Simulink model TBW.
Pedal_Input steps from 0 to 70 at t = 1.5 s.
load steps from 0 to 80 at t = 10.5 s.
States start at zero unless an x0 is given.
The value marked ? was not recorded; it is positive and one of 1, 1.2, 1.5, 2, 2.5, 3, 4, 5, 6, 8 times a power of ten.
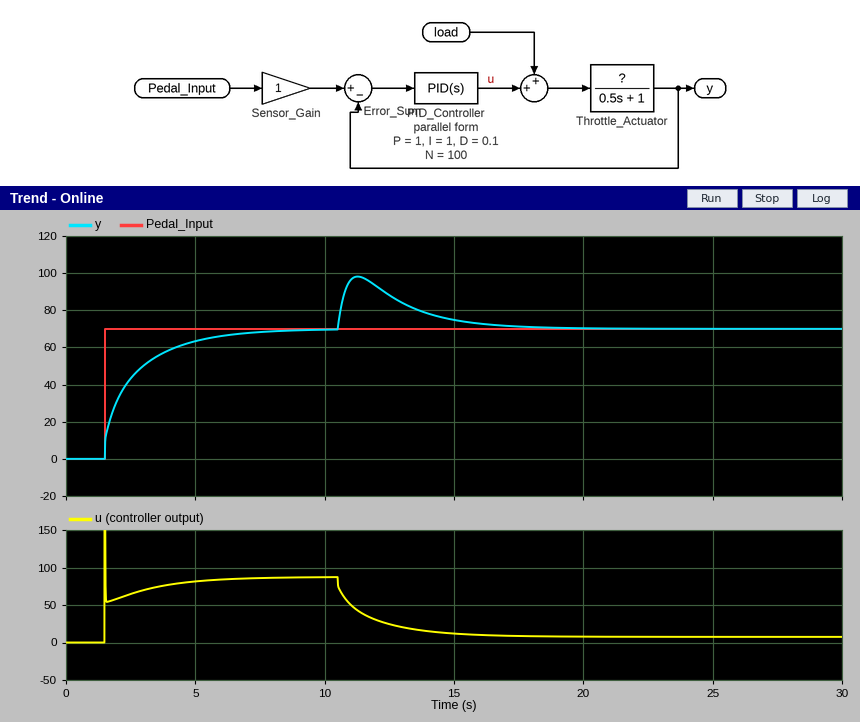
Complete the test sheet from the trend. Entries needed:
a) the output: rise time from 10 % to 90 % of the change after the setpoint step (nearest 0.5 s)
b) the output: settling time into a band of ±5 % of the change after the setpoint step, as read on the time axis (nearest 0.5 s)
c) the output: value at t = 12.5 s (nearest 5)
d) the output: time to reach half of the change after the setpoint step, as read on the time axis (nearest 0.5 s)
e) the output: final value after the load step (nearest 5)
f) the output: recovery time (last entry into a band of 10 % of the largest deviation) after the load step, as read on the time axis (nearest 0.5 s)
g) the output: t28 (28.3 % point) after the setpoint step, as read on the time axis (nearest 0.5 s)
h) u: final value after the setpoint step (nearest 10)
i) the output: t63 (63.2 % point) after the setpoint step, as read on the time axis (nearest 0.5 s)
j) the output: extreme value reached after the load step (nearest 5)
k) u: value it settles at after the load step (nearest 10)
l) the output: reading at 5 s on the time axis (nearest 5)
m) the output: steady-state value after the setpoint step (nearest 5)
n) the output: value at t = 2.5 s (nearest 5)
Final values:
3.5 s
6.0 s
90
2.0 s
70
16.0 s
1.5 s
90
2.5 s
100
10
65
70
45
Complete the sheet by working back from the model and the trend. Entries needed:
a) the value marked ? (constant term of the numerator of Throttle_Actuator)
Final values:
0.8
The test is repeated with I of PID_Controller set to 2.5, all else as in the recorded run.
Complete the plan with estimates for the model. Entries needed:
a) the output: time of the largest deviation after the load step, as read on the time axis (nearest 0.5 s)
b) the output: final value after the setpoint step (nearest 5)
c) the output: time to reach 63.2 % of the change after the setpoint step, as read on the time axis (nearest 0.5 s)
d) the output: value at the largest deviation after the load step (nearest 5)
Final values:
11.0 s
70
2.0 s
95
